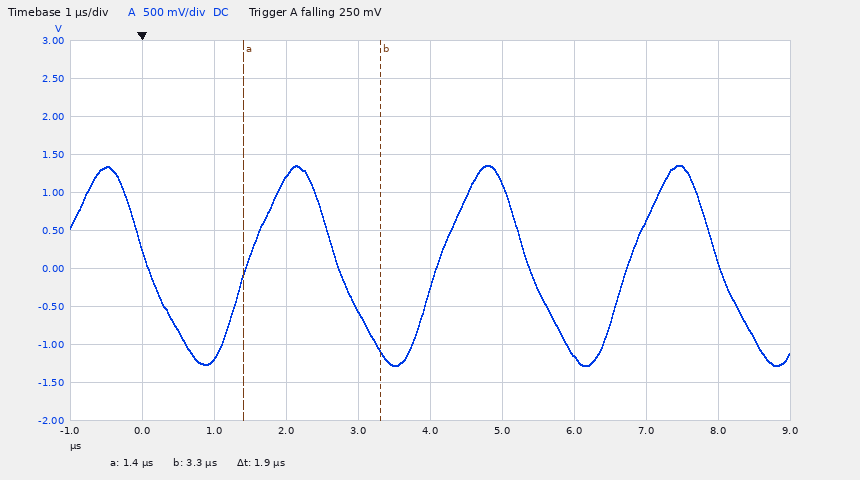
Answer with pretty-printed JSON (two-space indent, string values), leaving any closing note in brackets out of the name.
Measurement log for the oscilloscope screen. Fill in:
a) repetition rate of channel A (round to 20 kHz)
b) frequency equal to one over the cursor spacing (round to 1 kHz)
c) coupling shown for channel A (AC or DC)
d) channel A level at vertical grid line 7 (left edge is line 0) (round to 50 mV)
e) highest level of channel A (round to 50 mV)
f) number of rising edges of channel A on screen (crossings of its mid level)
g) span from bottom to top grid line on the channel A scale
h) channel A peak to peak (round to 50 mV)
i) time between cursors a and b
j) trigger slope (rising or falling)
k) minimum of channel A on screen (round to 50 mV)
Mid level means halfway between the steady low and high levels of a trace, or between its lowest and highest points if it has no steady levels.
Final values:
{
  "repetition rate of channel A": "380 kHz",
  "frequency equal to one over the cursor spacing": "526 kHz",
  "coupling shown for channel A": "DC",
  "channel A level at vertical grid line 7 (left edge is line 0)": "-1.15 V",
  "highest level of channel A": "1.35 V",
  "number of rising edges of channel A on screen": "3",
  "span from bottom to top grid line on the channel A scale": "5 V",
  "channel A peak to peak": "2.65 V",
  "time between cursors a and b": "1.9 µs",
  "trigger slope": "falling",
  "minimum of channel A on screen": "-1.30 V"
}
